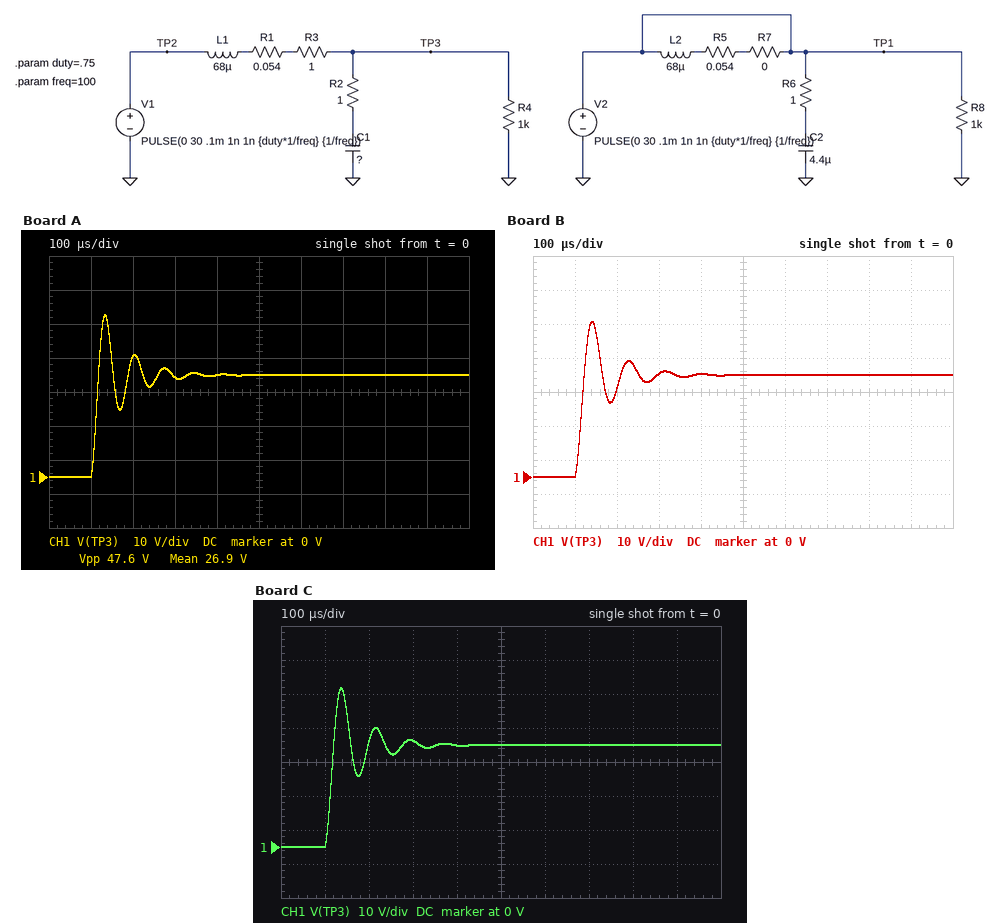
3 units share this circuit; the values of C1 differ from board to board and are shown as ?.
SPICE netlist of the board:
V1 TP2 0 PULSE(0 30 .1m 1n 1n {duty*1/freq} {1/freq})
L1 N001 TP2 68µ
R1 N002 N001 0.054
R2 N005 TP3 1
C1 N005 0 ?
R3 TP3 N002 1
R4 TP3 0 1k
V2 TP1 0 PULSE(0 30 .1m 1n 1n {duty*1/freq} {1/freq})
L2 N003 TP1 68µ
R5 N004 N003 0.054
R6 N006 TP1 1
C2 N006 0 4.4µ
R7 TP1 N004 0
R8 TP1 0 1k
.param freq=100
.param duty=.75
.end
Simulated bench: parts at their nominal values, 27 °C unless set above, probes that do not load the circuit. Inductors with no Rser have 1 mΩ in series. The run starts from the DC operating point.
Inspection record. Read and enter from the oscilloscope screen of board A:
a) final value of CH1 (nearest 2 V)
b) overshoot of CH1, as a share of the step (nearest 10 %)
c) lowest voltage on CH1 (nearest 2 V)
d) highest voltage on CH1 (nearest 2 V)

30 V
60 %
0 V
48 V
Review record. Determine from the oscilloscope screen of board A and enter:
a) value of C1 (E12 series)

1.8 µF
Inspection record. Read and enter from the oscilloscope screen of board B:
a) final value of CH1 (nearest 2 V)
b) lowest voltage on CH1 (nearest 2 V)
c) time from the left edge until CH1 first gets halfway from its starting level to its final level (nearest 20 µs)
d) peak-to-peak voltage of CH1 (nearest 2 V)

30 V
0 V
120 µs
46 V
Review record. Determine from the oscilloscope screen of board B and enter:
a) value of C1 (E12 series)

2.7 µF
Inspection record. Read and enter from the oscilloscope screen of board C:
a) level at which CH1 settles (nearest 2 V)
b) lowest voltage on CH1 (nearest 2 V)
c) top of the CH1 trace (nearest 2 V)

30 V
0 V
46 V
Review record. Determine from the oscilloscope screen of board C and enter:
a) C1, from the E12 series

2.2 µF
